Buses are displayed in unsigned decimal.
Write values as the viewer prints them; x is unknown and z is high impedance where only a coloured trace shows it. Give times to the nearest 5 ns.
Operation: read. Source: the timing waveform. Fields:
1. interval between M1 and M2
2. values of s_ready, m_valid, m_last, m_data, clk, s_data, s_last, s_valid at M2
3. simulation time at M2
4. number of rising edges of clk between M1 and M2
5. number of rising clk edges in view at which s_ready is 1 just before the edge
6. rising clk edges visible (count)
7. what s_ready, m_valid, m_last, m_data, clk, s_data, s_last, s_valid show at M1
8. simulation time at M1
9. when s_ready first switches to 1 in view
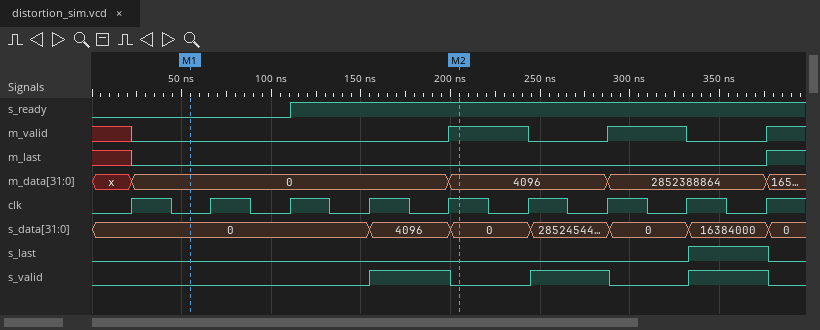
150 ns
s_ready=1, m_valid=1, m_last=0, m_data=4096, clk=1, s_data=0, s_last=0, s_valid=0
205 ns
4
6
9
s_ready=0, m_valid=0, m_last=0, m_data=0, clk=0, s_data=0, s_last=0, s_valid=0
55 ns
110 ns
